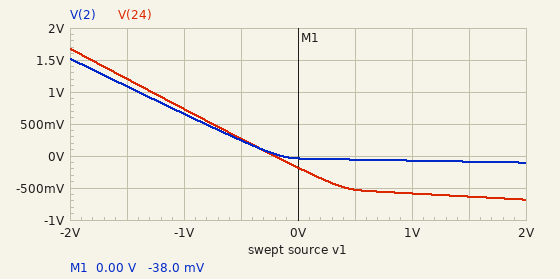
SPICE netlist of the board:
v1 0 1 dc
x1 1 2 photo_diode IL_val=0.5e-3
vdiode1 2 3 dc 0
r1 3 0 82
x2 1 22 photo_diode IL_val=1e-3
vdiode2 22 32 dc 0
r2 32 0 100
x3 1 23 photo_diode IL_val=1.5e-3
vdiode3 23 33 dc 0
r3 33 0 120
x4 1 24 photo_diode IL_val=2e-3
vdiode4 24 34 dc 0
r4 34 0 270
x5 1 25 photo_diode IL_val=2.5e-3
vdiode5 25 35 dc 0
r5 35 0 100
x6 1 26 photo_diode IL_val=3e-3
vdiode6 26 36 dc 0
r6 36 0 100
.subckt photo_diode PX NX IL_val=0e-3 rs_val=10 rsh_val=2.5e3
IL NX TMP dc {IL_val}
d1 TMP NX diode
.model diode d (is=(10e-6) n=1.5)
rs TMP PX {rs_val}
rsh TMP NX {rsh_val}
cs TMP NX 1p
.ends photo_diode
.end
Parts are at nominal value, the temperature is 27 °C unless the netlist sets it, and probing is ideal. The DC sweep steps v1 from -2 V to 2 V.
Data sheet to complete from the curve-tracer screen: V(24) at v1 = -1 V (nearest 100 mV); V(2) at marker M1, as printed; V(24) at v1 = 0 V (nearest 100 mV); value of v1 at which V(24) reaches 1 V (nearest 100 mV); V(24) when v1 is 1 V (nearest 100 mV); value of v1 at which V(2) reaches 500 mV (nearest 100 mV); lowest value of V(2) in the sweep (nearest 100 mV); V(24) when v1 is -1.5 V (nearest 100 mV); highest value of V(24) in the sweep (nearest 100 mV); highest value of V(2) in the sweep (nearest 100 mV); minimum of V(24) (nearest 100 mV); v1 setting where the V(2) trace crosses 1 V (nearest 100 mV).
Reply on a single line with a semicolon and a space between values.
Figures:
700 mV; -38.0 mV; -200 mV; -1.3 V; -600 mV; -800 mV; -100 mV; 1.2 V; 1.7 V; 1.5 V; -700 mV; -1.4 V
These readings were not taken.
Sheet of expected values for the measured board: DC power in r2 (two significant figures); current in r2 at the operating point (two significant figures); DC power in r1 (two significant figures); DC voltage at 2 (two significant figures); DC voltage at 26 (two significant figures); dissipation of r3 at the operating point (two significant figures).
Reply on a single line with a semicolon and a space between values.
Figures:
74 µW; 860 µA; 18 µW; -38 mV; -170 mV; 140 µW
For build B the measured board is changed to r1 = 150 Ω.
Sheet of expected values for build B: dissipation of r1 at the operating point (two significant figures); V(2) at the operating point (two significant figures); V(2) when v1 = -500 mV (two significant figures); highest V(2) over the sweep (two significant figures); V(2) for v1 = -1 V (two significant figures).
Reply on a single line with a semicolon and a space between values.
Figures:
27 µW; -64 mV; 270 mV; 1.6 V; 710 mV
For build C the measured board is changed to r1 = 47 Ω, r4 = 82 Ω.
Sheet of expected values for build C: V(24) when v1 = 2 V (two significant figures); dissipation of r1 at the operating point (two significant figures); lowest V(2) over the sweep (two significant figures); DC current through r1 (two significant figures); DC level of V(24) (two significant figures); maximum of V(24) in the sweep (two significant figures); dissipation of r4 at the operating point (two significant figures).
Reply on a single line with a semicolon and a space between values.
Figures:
-220 mV; 11 µW; -60 mV; 480 µA; -130 mV; 1.5 V; 200 µW
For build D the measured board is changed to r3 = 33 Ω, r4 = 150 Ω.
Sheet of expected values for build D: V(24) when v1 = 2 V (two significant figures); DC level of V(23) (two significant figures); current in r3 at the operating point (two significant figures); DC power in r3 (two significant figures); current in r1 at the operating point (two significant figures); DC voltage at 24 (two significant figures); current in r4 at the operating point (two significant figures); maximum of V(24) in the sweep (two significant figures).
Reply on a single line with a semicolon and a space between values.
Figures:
-400 mV; -47 mV; 1.4 mA; 68 µW; 460 µA; -160 mV; 1.1 mA; 1.6 V
